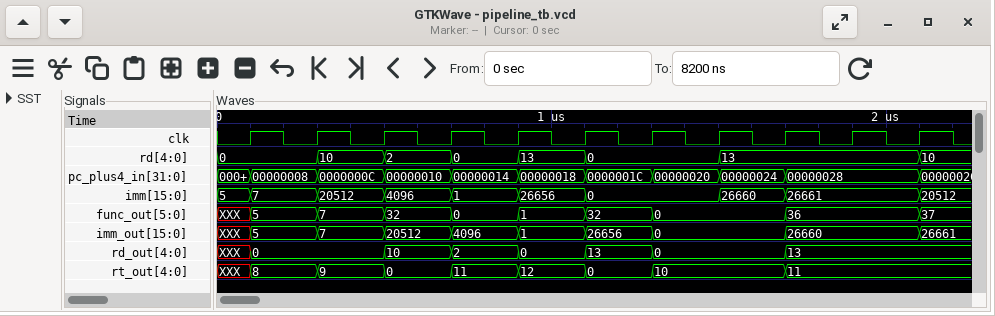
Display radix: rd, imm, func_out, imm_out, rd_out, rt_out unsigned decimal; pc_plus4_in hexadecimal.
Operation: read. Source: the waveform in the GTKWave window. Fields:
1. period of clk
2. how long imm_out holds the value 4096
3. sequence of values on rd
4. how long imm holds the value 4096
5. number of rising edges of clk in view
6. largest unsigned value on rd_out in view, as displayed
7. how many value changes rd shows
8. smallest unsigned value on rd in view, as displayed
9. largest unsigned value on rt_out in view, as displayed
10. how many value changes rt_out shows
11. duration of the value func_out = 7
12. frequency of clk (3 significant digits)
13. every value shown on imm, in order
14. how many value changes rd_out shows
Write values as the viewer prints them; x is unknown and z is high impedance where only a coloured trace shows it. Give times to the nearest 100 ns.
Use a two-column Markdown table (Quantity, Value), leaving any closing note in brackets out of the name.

| Quantity | Value |
|---|---|
| period of clk | 200 ns |
| how long imm_out holds the value 4096 | 200 ns |
| sequence of values on rd | 0, 10, 2, 0, 13, 0, 13, 10 |
| how long imm holds the value 4096 | 200 ns |
| number of rising edges of clk in view | 11 |
| largest unsigned value on rd_out in view, as displayed | 13 |
| how many value changes rd shows | 7 |
| smallest unsigned value on rd in view, as displayed | 0 |
| largest unsigned value on rt_out in view, as displayed | 12 |
| how many value changes rt_out shows | 8 |
| duration of the value func_out = 7 | 200 ns |
| frequency of clk | 5.00 MHz |
| every value shown on imm, in order | 5, 7, 20512, 4096, 1, 26656, 0, 26660, 26661, 20512 |
| how many value changes rd_out shows | 7 |
